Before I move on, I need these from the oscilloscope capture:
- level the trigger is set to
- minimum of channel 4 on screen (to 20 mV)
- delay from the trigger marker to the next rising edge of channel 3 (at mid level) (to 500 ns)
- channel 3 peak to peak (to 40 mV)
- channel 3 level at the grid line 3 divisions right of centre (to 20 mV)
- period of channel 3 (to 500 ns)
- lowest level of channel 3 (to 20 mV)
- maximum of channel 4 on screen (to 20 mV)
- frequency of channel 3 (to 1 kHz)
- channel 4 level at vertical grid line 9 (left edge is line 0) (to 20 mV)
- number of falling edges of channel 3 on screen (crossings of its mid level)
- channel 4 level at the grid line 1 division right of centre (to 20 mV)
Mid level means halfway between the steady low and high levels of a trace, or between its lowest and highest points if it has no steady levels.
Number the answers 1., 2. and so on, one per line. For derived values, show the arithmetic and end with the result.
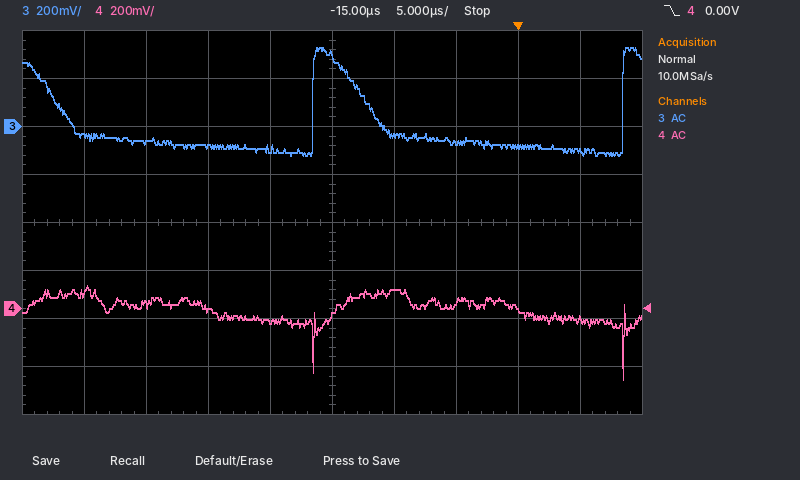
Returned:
1. 0.00 V
2. -300 mV
3. 8.5 µs
4. 440 mV
5. -80 mV
6. 25.0 µs
7. -120 mV
8. 100 mV
9. 1 / 25.0 µs ≈ 40 kHz
10. -40 mV
11. 2
12. 80 mV
